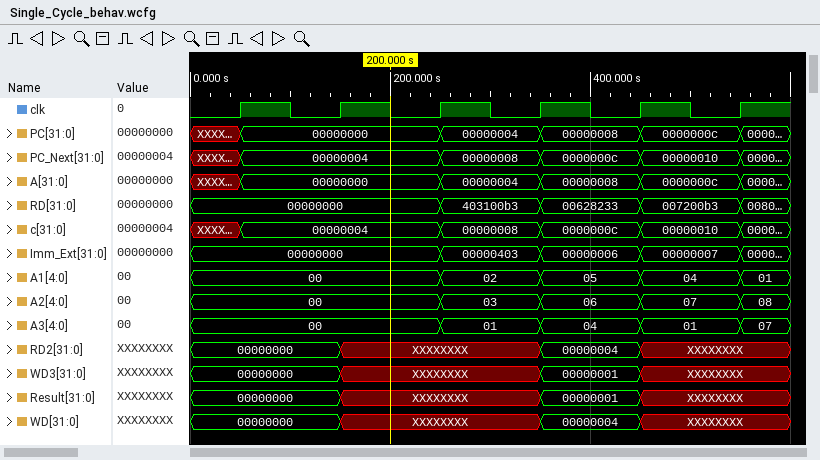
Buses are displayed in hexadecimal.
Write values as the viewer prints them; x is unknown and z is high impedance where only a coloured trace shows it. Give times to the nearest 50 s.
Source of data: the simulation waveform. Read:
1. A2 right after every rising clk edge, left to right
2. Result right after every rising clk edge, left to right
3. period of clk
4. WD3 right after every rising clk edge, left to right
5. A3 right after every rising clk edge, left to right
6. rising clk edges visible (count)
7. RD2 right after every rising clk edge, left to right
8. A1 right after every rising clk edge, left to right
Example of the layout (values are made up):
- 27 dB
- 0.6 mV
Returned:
- 00, 00, 03, 06, 07, 08
- 00000000, XXXXXXXX, XXXXXXXX, 00000001, XXXXXXXX, XXXXXXXX
- 100 s
- 00000000, XXXXXXXX, XXXXXXXX, 00000001, XXXXXXXX, XXXXXXXX
- 00, 00, 01, 04, 01, 07
- 6
- 00000000, XXXXXXXX, XXXXXXXX, 00000004, XXXXXXXX, XXXXXXXX
- 00, 00, 02, 05, 04, 01
